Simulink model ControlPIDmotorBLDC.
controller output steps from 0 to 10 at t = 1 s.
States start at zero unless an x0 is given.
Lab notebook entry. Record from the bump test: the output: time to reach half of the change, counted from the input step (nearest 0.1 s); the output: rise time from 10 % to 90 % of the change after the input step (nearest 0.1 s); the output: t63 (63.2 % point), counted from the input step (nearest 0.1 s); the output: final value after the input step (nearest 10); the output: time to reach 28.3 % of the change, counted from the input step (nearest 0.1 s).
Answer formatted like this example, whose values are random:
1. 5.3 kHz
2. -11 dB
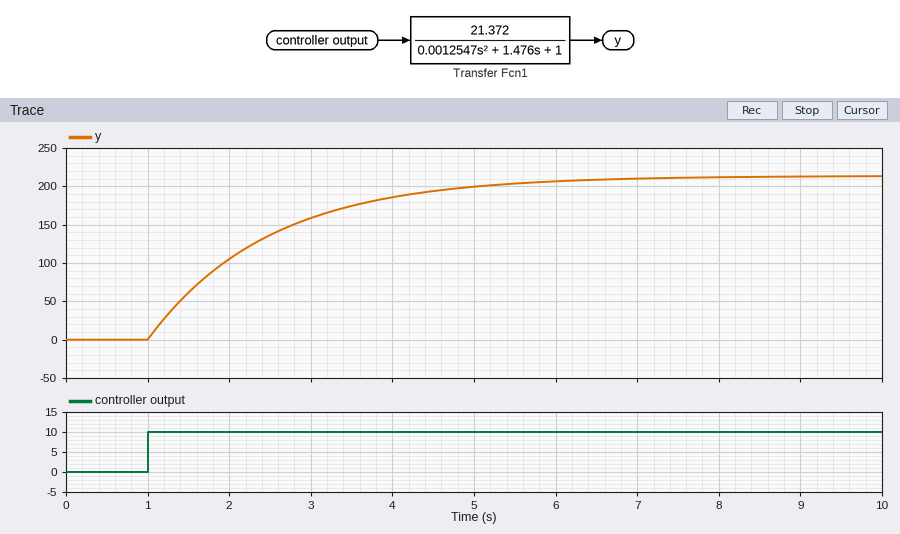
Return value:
1. 1.0 s
2. 3.2 s
3. 1.5 s
4. 210
5. 0.5 s
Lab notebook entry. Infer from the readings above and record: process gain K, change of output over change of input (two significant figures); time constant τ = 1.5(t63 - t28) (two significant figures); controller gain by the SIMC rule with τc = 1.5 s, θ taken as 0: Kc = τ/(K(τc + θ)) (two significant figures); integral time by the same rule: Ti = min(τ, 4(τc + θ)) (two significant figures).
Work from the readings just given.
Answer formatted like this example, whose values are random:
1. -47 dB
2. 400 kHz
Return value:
1. 21
2. 1.5 s
3. 0.048
4. 1.5 s
